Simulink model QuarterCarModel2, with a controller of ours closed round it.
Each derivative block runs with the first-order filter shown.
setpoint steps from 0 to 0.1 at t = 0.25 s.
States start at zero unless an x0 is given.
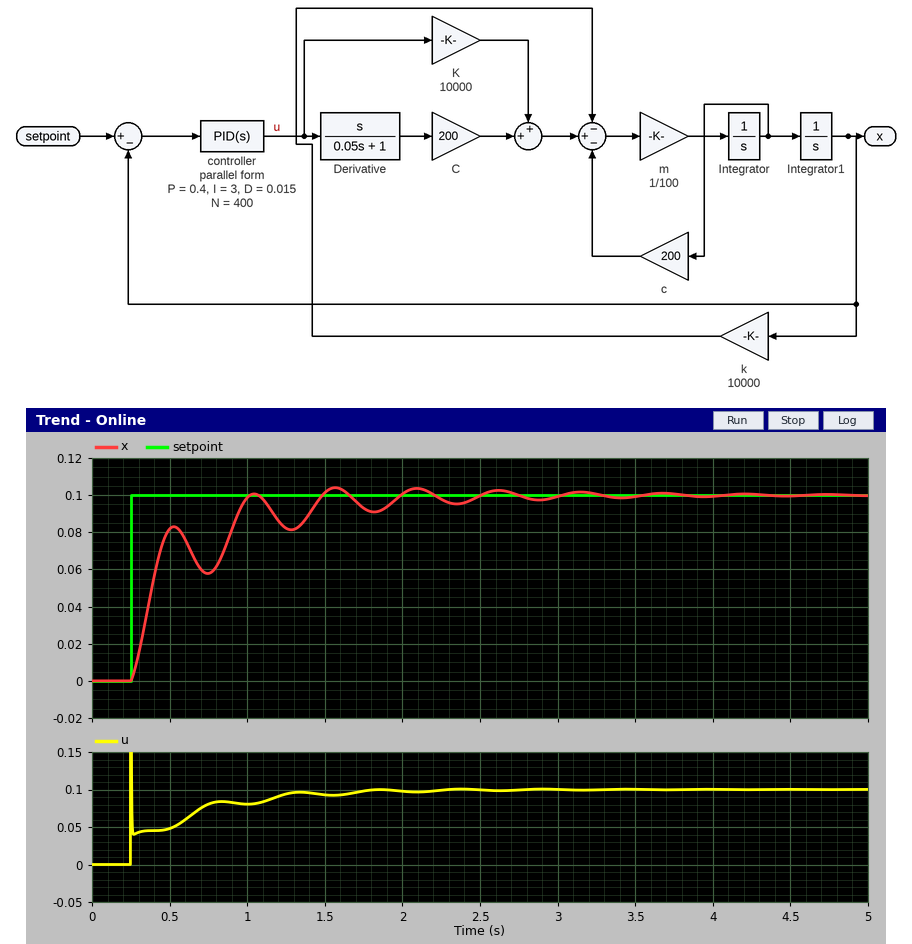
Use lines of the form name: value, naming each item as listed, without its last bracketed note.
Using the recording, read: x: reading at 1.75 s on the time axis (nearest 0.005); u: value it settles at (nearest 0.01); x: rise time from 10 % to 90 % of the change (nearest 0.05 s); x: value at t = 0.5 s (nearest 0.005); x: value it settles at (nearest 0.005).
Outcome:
x: reading at 1.75 s on the time axis: 0.095
u: value it settles at: 0.10
x: rise time from 10 % to 90 % of the change: 0.65 s
x: value at t = 0.5 s: 0.080
x: value it settles at: 0.100
